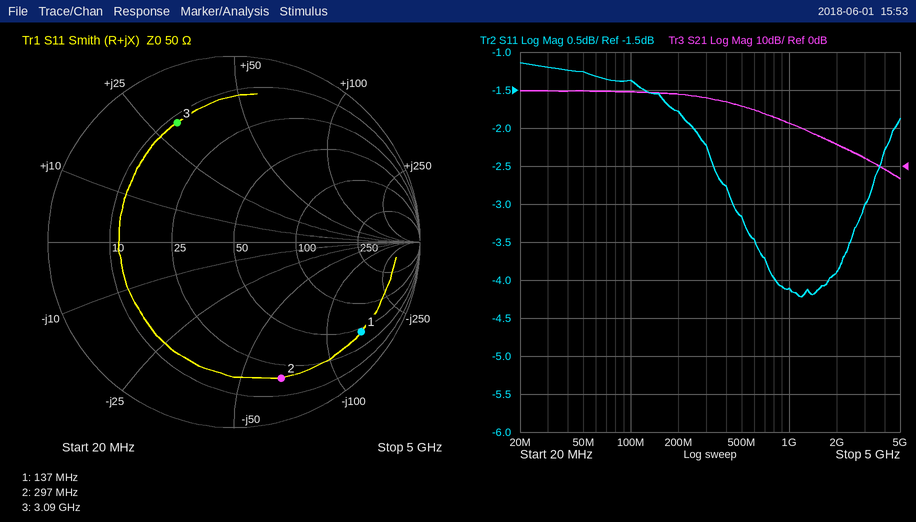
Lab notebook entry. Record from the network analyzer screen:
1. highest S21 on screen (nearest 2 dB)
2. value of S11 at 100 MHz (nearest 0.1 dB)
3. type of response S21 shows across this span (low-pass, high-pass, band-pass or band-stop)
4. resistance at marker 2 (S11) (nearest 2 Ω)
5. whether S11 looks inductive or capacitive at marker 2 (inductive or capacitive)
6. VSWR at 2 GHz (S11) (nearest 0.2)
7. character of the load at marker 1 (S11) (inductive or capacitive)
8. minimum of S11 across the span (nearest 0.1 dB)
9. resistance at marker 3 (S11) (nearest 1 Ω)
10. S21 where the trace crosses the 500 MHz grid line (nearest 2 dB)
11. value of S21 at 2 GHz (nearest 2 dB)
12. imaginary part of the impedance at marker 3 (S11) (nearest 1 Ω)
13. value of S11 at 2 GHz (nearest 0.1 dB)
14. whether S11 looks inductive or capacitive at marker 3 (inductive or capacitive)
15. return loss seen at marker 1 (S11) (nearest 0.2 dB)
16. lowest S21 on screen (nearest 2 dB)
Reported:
20 dB
-1.4 dB
low-pass
18 Ω
capacitive
4.6
capacitive
-4.2 dB
12 Ω
16 dB
6 dB
+30 Ω
-3.9 dB
inductive
1.6 dB
-4 dB
